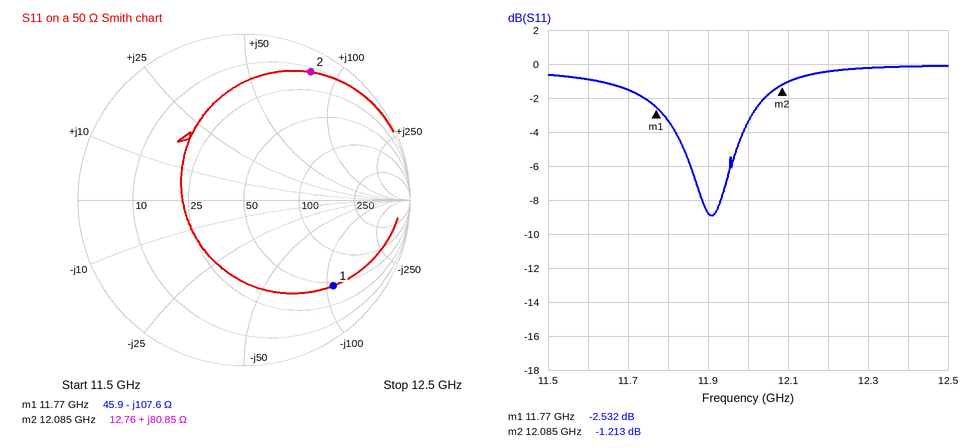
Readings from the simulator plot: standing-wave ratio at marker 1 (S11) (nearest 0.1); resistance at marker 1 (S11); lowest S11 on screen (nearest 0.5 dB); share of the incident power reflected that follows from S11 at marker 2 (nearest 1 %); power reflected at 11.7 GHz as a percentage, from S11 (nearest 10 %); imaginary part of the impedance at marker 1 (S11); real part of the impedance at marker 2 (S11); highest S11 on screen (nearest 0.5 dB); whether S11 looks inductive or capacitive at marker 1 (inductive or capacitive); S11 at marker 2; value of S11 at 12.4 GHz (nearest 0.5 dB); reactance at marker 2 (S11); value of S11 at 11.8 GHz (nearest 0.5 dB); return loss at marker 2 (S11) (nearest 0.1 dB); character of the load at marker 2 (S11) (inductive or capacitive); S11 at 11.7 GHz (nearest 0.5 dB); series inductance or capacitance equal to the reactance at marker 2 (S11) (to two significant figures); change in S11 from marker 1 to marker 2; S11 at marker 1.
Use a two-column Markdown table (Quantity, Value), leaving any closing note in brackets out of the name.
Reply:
| Quantity | Value |
|---|---|
| standing-wave ratio at marker 1 (S11) | 6.9 |
| resistance at marker 1 | 45.9 Ω |
| lowest S11 on screen | -9.0 dB |
| share of the incident power reflected that follows from S11 at marker 2 | 76 % |
| power reflected at 11.7 GHz as a percentage, from S11 | 70 % |
| imaginary part of the impedance at marker 1 | -107.6 Ω |
| real part of the impedance at marker 2 | 12.76 Ω |
| highest S11 on screen | 0.0 dB |
| whether S11 looks inductive or capacitive at marker 1 | capacitive |
| S11 at marker 2 | -1.213 dB |
| value of S11 at 12.4 GHz | 0.0 dB |
| reactance at marker 2 | +80.85 Ω |
| value of S11 at 11.8 GHz | -3.5 dB |
| return loss at marker 2 (S11) | 1.2 dB |
| character of the load at marker 2 (S11) | inductive |
| S11 at 11.7 GHz | -1.5 dB |
| series inductance or capacitance equal to the reactance at marker 2 (S11) | 1.1 nH |
| change in S11 from marker 1 to marker 2 | 1.319 dB |
| S11 at marker 1 | -2.532 dB |
